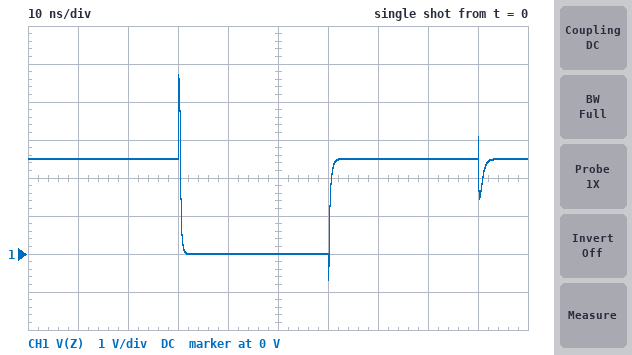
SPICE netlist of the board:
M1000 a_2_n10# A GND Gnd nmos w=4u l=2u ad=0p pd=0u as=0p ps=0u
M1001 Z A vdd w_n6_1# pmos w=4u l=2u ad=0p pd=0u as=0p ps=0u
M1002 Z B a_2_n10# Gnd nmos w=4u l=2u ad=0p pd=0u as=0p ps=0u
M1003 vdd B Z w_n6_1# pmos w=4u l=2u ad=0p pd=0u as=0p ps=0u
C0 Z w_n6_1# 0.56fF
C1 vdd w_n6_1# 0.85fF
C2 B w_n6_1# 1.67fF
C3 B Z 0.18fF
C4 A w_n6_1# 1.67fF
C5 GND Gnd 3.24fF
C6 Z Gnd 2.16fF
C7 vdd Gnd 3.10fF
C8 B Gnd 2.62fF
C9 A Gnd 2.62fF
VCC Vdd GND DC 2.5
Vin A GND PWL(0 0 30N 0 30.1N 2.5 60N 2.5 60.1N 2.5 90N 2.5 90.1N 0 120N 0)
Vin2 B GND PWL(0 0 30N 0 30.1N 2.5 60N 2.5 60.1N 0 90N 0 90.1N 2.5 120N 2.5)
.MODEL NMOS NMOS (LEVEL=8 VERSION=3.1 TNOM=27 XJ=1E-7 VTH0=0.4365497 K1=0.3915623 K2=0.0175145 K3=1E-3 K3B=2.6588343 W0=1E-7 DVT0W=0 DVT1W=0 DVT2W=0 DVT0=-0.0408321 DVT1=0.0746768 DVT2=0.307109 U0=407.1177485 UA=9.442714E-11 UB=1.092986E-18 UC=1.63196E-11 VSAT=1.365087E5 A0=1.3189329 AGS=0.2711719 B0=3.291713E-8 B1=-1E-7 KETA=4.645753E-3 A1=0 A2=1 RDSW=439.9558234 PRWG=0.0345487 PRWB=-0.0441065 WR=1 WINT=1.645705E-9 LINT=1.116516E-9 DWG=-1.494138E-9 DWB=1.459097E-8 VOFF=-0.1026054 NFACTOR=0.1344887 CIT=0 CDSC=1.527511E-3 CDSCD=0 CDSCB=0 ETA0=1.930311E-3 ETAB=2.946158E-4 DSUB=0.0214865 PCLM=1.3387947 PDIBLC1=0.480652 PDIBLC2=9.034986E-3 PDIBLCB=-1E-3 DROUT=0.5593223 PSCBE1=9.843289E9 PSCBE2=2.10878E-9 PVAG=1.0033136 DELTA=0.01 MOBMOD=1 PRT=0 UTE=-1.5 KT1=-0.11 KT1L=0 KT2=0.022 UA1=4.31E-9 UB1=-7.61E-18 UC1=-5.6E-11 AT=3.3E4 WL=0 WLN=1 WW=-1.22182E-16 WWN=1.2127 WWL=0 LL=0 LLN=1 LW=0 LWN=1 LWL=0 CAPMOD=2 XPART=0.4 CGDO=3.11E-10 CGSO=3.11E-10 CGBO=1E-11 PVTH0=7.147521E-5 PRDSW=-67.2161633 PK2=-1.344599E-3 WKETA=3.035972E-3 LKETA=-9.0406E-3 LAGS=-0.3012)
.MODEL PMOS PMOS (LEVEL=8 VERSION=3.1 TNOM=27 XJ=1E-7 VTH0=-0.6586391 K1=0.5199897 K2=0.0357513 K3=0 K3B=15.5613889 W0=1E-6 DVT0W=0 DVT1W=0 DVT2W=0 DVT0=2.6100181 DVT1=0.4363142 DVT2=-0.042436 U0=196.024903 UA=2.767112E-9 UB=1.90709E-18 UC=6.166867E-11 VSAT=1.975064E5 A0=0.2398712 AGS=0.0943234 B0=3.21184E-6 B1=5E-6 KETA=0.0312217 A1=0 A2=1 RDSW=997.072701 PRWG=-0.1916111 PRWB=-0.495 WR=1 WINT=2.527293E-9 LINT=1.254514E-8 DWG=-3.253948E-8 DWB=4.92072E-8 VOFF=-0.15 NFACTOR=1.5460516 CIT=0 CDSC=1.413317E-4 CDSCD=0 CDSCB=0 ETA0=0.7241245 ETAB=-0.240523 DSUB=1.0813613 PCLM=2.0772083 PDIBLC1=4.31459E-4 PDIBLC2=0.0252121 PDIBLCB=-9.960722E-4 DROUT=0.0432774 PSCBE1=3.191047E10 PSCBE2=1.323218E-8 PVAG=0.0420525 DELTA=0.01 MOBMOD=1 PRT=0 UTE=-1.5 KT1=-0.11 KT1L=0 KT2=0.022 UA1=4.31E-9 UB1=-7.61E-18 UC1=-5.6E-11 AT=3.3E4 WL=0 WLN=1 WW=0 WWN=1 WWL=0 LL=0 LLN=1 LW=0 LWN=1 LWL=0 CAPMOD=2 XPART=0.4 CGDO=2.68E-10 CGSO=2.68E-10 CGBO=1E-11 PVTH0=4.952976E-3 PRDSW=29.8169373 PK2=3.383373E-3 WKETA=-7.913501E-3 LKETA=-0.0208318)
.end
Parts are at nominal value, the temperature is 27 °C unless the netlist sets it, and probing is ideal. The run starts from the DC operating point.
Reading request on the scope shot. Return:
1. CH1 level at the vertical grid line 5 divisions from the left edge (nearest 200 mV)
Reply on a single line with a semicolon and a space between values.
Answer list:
0 V
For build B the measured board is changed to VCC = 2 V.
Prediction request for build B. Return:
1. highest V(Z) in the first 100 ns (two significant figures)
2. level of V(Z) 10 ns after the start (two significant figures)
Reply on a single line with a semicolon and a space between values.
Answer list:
4.3 V; 2.0 V
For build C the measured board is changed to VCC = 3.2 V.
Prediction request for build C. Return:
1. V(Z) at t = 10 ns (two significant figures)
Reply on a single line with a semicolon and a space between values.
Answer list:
3.2 V
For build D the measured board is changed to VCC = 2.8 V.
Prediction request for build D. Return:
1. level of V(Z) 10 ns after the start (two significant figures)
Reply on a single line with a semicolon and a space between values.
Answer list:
2.8 V
